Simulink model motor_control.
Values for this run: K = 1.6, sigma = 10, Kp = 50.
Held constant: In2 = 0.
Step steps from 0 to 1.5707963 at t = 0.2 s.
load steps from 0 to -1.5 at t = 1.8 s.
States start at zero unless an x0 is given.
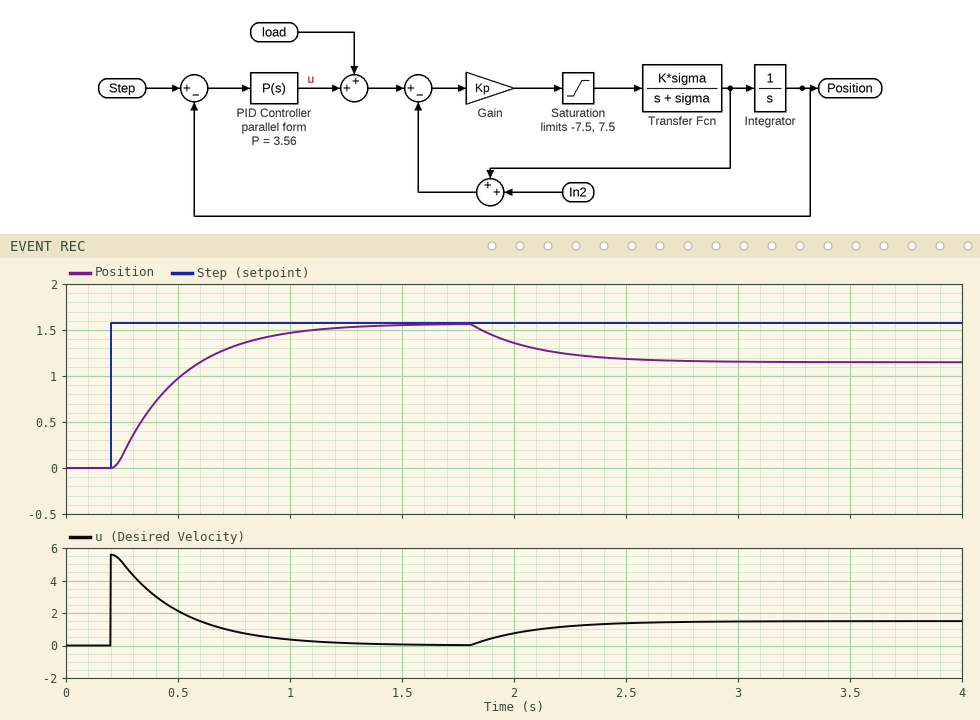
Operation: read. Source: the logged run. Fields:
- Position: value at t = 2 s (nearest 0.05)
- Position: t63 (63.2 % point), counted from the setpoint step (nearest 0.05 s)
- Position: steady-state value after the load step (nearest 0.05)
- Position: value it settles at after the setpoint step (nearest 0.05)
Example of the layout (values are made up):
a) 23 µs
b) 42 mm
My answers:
a) 1.35
b) 0.30 s
c) 1.15
d) 1.55
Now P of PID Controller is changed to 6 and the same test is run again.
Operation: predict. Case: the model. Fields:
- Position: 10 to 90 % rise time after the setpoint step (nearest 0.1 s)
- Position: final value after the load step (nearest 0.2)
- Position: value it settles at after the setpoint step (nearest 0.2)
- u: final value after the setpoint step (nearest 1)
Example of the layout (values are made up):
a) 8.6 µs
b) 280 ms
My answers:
a) 0.4 s
b) 1.4
c) 1.6
d) 0
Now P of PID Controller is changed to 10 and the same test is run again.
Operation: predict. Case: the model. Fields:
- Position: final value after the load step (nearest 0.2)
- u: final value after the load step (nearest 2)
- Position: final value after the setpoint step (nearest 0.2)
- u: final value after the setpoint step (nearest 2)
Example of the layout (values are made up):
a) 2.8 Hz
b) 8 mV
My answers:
a) 1.4
b) 2
c) 1.6
d) 0
